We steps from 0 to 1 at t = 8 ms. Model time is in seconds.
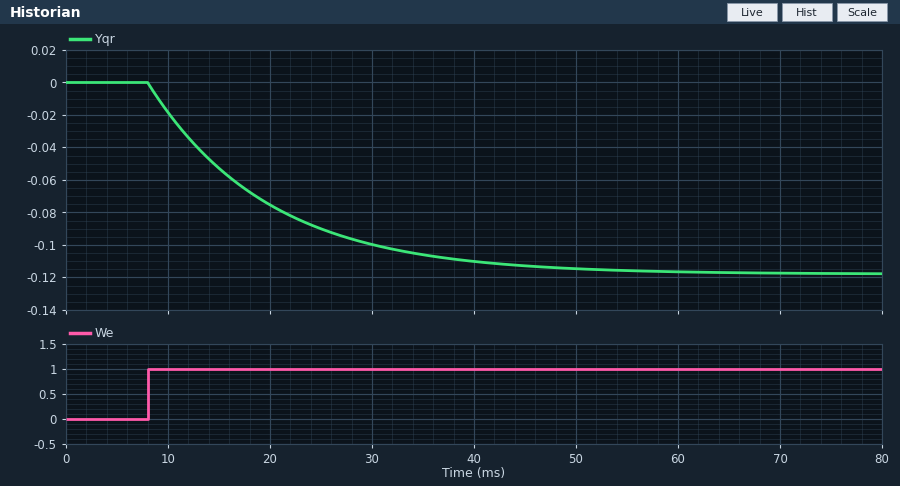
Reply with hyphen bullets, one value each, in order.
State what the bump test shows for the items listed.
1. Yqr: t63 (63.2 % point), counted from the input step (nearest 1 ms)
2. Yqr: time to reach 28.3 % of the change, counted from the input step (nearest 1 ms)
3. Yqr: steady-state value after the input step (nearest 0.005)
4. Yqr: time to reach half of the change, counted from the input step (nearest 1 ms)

- 12 ms
- 4 ms
- -0.120
- 8 ms
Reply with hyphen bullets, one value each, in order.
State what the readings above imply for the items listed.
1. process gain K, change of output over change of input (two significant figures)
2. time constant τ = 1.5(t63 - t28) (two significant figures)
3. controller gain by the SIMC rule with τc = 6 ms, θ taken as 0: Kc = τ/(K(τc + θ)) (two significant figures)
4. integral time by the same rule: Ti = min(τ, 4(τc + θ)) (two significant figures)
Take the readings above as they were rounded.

- -0.12
- 12 ms
- -17
- 12 ms
